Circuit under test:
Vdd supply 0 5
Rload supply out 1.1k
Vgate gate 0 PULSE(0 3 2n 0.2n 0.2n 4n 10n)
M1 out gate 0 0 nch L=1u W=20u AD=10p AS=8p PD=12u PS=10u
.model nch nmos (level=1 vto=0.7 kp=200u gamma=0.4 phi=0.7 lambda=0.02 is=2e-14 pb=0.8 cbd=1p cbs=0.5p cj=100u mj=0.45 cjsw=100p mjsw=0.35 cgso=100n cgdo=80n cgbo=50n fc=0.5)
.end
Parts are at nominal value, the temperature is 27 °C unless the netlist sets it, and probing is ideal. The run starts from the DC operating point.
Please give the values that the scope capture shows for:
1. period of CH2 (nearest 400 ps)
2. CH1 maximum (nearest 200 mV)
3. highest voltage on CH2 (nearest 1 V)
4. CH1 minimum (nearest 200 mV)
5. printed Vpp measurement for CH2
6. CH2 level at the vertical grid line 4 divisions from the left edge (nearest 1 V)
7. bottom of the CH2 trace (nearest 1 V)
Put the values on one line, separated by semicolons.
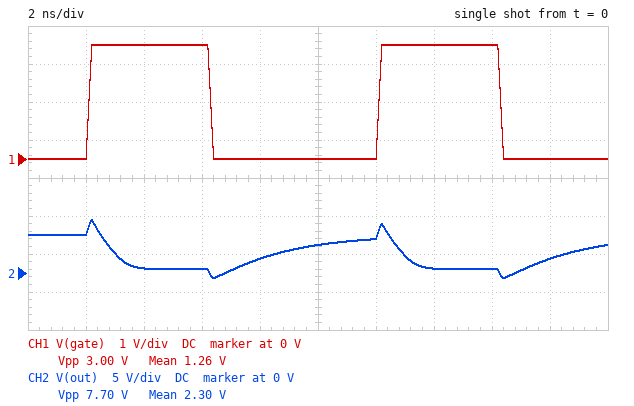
10.0 ns; 3.0 V; 7 V; 0 V; 7.70 V; 2 V; -1 V
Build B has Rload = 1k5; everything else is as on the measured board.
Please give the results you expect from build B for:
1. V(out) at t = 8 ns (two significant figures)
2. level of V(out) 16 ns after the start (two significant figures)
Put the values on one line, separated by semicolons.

1.3 V; 360 mV
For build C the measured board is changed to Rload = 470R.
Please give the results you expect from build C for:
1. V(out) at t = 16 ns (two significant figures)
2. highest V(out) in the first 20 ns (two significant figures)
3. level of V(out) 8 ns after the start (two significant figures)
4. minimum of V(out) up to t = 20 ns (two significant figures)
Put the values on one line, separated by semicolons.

1.2 V; 6.9 V; 3.9 V; -170 mV
